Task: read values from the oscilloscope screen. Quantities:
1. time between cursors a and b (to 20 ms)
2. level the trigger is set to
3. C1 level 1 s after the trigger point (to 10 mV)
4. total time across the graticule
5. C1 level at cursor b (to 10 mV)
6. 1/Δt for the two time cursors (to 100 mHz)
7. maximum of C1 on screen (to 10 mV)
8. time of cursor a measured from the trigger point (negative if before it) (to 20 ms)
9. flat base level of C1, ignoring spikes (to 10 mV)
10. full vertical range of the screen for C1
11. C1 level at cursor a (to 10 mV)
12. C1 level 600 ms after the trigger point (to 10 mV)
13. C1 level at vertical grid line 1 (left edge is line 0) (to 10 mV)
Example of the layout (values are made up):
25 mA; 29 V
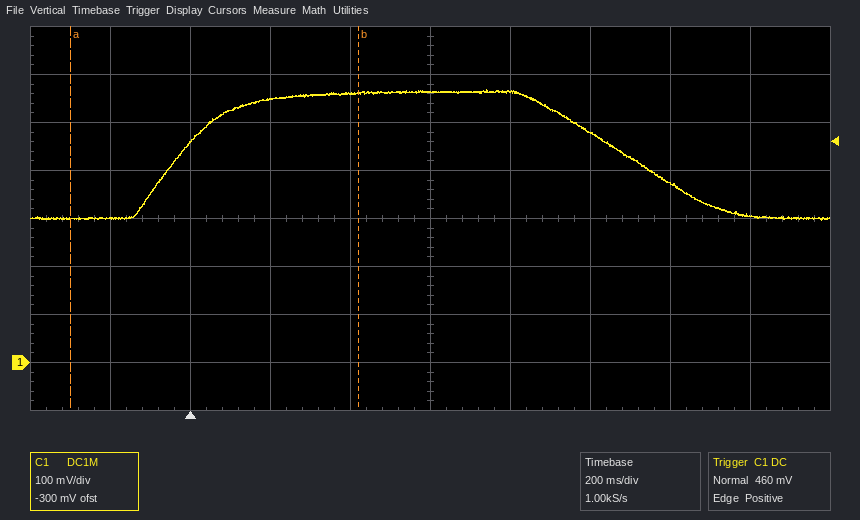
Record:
720 ms; 460 mV; 480 mV; 2 s; 560 mV; 1.4 Hz; 570 mV; -300 ms; 300 mV; 800 mV; 300 mV; 560 mV; 300 mV
